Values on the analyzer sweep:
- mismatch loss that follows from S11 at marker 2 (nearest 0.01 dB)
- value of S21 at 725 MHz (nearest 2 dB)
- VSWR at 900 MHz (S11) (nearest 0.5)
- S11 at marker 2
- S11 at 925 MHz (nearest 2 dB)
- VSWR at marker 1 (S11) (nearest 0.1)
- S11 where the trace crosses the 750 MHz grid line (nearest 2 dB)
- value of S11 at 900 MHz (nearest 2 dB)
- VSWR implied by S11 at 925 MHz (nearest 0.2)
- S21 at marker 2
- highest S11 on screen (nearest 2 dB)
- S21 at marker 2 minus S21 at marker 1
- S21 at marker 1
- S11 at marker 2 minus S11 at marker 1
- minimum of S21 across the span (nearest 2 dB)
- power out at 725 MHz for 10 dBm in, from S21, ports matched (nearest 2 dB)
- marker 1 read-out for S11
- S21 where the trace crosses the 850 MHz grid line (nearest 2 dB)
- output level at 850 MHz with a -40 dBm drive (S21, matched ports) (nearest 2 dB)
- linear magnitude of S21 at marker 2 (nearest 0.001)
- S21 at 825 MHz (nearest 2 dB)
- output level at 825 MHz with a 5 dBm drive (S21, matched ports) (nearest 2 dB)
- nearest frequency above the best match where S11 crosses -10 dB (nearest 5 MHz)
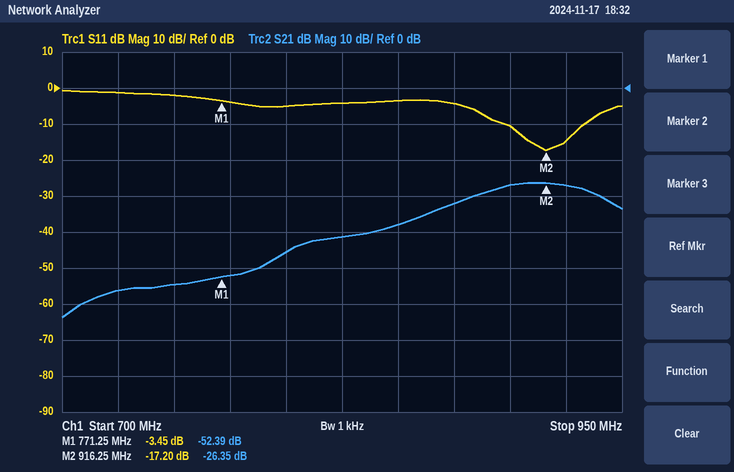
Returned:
0.08 dB
-56 dB
2.0
-17.20 dB
-14 dB
5.1
-2 dB
-10 dB
1.4
-26.35 dB
0 dB
26.04 dB
-52.39 dB
-13.75 dB
-64 dB
-46 dBm
-3.45 dB
-38 dB
-78 dBm
0.048
-42 dB
-36 dBm
935 MHz
